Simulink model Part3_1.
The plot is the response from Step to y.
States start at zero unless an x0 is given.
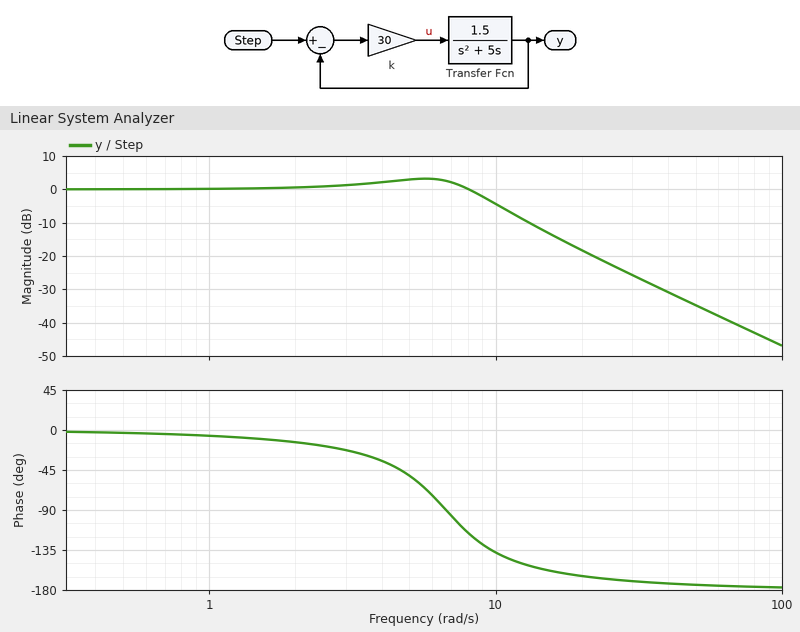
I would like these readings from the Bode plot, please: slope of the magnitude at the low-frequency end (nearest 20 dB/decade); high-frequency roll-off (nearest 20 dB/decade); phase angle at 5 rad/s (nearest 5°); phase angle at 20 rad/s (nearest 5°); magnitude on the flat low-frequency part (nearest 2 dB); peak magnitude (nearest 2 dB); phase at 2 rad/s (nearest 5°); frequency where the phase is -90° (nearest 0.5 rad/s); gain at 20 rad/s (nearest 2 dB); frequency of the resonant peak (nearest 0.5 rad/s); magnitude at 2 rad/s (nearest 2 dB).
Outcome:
0 dB/decade
-40 dB/decade
-50°
-165°
0 dB
4 dB
-15°
6.5 rad/s
-18 dB
5.5 rad/s
0 dB
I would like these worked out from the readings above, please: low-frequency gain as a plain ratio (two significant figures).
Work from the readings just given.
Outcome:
1.0
